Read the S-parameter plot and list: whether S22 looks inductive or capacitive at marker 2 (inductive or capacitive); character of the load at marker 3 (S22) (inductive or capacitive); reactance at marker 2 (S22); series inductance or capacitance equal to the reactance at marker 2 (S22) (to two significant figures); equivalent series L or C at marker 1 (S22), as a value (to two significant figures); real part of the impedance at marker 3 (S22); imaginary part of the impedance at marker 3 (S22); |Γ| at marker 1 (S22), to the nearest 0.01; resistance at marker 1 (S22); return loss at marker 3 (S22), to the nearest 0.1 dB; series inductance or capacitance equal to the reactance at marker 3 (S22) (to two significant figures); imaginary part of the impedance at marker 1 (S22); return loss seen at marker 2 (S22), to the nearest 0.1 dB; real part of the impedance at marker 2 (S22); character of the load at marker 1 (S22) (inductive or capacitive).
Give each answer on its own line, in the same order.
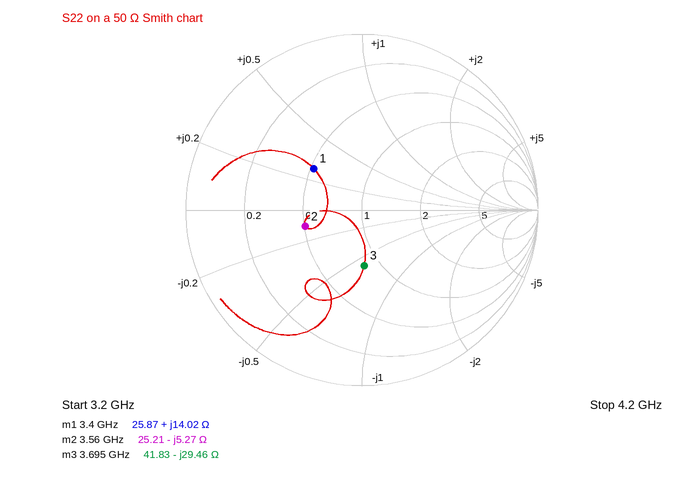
capacitive
capacitive
-5.27 Ω
8.5 pF
660 pH
41.83 Ω
-29.46 Ω
0.36
25.87 Ω
10.0 dB
1.5 pF
+14.02 Ω
9.5 dB
25.21 Ω
inductive
